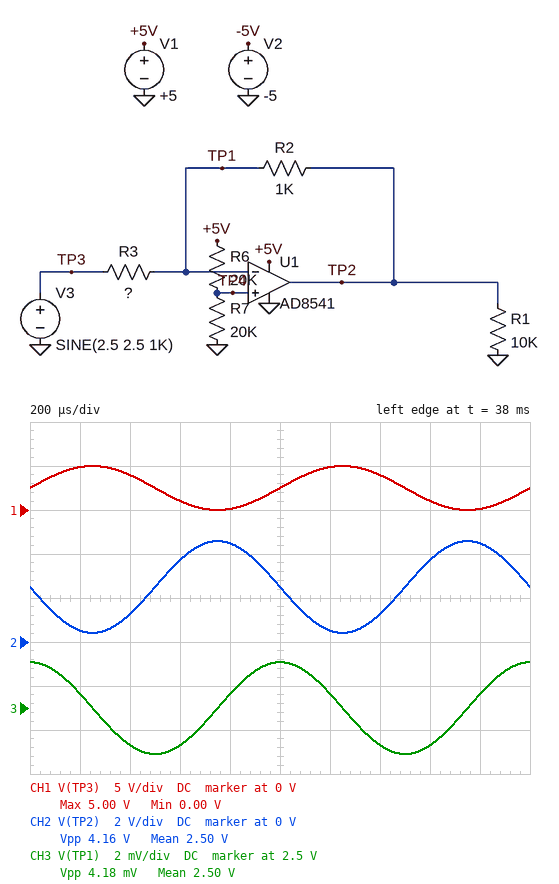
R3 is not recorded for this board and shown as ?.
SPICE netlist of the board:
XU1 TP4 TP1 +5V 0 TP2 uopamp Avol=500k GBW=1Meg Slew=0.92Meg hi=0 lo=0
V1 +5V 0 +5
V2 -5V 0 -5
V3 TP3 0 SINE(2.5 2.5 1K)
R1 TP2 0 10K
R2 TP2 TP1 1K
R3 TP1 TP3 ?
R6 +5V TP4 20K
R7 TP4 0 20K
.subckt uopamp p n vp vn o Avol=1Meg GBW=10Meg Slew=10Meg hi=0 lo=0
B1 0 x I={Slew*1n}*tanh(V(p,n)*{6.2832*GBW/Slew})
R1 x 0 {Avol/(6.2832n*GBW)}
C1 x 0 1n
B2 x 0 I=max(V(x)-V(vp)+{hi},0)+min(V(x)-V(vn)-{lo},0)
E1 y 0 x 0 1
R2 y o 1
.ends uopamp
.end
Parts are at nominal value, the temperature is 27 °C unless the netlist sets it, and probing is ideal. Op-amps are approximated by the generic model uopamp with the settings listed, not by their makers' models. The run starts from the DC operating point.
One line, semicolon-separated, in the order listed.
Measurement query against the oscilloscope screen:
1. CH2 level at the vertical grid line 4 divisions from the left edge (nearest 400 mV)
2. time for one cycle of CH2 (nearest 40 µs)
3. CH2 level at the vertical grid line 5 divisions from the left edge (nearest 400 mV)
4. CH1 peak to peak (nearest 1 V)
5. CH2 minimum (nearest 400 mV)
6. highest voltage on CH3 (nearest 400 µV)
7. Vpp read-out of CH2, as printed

4.4 V; 1.00 ms; 2.4 V; 5 V; 400 mV; 2.5020 V; 4.16 V
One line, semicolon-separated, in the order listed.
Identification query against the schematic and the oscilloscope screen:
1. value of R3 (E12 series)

1.2 kΩ
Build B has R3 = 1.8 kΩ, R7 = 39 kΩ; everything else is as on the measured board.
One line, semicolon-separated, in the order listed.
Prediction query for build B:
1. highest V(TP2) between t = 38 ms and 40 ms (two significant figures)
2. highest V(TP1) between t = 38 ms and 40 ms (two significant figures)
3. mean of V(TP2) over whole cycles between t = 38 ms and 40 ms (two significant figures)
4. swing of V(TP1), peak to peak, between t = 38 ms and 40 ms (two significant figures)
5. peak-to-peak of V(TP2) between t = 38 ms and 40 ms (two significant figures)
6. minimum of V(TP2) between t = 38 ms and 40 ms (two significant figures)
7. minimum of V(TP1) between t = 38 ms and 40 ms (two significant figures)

5.0 V; 3.3 V; 3.7 V; 93 mV; 2.6 V; 2.4 V; 3.2 V
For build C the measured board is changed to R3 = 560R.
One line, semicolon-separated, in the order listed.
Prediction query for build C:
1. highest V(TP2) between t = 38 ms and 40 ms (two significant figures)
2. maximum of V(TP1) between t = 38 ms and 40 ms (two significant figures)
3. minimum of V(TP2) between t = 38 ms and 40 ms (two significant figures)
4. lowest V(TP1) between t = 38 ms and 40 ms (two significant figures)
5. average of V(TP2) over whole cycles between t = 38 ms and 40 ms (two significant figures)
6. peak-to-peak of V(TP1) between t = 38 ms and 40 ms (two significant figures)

5.0 V; 3.2 V; 1.9 mV; 1.8 V; 2.5 V; 1.4 V
